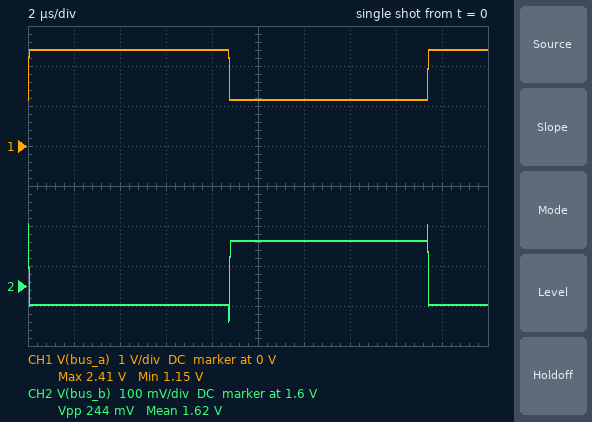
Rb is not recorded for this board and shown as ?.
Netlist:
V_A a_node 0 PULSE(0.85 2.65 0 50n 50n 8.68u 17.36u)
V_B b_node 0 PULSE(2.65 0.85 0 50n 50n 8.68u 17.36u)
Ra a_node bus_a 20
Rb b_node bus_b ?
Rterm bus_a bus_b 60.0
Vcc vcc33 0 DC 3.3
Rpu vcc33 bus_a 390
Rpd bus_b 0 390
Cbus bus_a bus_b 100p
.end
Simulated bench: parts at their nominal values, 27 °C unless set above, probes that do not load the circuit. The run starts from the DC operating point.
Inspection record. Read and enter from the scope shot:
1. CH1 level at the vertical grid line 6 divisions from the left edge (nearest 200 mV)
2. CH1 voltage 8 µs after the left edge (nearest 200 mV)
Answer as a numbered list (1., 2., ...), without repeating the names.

1. 1.2 V
2. 2.4 V
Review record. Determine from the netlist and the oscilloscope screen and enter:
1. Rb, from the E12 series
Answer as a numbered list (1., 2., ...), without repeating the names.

1. 68 Ω
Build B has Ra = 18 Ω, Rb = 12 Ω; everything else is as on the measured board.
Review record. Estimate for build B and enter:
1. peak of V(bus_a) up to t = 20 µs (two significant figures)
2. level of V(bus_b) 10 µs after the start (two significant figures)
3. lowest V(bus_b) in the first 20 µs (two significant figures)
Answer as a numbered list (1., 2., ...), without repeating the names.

1. 2.3 V
2. 2.4 V
3. 1.1 V
